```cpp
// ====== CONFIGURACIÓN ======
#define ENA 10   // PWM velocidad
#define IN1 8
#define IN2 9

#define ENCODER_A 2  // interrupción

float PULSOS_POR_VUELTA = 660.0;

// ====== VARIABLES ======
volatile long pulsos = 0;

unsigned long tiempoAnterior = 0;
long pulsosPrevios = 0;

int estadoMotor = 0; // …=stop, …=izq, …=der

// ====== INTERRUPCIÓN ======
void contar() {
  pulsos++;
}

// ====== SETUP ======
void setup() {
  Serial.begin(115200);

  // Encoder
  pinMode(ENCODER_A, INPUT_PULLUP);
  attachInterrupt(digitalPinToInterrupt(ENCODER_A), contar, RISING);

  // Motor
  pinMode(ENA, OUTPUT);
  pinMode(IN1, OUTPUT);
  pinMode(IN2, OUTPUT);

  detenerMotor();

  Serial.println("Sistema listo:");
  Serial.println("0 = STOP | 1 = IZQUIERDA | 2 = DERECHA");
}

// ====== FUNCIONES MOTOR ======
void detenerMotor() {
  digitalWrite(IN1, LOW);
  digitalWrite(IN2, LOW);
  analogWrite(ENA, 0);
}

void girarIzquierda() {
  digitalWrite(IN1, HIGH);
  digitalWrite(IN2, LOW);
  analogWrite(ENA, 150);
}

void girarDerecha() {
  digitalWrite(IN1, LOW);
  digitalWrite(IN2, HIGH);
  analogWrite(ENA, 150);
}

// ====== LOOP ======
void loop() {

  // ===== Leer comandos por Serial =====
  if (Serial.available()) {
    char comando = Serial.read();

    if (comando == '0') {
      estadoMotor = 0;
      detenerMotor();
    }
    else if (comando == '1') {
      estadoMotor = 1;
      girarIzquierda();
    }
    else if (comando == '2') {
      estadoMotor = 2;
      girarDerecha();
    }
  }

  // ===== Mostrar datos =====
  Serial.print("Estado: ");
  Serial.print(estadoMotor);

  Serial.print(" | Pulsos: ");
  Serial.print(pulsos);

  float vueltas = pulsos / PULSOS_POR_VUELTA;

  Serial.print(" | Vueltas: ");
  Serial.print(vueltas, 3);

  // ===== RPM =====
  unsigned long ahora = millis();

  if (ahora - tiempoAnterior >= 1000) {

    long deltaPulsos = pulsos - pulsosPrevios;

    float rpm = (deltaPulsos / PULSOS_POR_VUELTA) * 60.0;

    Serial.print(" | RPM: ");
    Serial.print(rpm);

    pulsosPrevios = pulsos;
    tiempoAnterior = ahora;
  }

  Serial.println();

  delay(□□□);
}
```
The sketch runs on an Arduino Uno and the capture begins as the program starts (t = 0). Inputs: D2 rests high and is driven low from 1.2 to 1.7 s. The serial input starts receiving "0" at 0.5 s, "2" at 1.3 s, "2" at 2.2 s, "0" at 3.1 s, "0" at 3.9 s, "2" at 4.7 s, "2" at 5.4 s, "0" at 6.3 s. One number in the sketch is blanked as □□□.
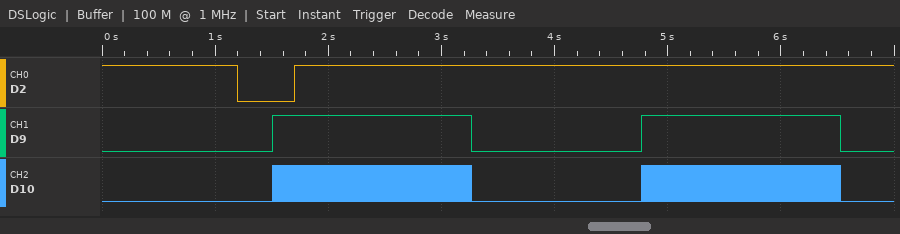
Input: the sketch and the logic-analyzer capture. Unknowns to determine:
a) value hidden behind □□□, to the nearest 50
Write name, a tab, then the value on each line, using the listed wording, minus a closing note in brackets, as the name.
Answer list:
value hidden behind □□□, to the nearest 50	250
